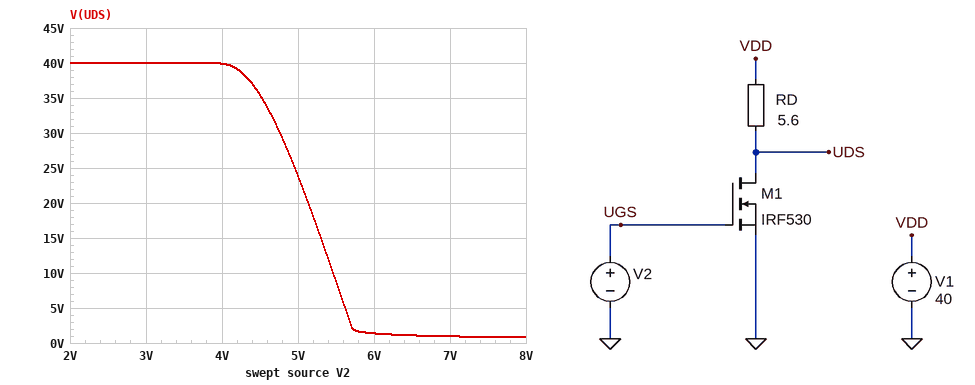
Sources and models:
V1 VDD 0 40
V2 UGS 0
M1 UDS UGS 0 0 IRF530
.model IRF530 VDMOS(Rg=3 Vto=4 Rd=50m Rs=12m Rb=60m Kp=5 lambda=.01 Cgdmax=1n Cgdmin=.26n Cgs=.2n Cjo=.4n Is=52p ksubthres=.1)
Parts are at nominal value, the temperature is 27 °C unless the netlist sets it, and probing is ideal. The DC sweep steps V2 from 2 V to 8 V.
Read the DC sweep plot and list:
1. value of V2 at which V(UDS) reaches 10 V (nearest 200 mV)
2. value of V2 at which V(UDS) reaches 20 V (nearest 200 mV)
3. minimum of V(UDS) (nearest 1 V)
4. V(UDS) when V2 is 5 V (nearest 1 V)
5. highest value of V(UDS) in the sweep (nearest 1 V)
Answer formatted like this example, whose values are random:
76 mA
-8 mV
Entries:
5.4 V
5.2 V
1 V
24 V
40 V
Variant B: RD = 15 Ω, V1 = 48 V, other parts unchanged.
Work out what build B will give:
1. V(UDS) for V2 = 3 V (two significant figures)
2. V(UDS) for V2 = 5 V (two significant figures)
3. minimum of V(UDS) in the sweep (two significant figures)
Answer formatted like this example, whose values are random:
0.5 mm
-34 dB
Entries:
48 V
9.5 V
360 mV
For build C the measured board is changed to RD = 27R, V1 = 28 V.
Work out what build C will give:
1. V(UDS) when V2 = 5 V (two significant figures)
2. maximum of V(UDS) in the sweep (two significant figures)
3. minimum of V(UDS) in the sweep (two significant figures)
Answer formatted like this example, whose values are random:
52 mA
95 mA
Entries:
300 mV
28 V
120 mV
